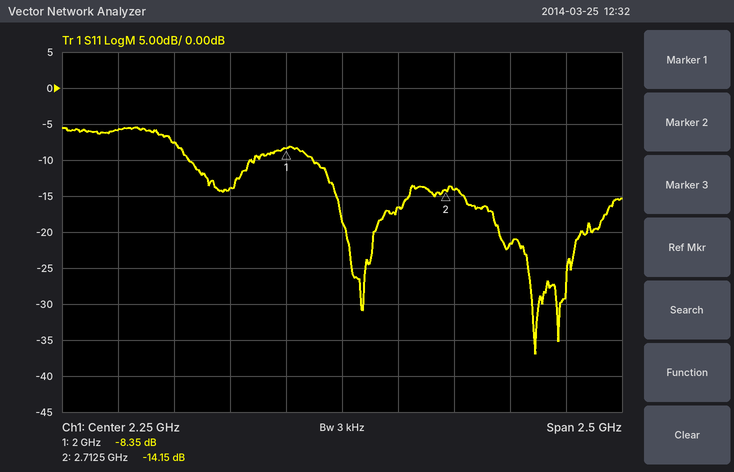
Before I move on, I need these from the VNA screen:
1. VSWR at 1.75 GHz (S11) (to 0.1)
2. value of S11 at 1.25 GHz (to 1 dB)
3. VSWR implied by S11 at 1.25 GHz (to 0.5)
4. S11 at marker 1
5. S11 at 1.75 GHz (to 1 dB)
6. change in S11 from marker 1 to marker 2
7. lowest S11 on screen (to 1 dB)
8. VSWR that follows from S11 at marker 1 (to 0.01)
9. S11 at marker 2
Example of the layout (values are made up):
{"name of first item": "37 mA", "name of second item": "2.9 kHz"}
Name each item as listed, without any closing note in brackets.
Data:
{"VSWR at 1.75 GHz (S11)": "1.5", "value of S11 at 1.25 GHz": "-6 dB", "VSWR implied by S11 at 1.25 GHz": "3.0", "S11 at marker 1": "-8.35 dB", "S11 at 1.75 GHz": "-14 dB", "change in S11 from marker 1 to marker 2": "-5.80 dB", "lowest S11 on screen": "-37 dB", "VSWR that follows from S11 at marker 1": "2.24", "S11 at marker 2": "-14.15 dB"}
